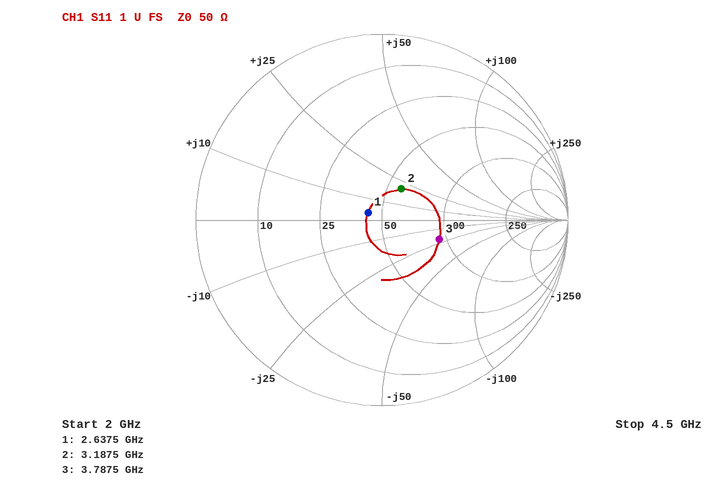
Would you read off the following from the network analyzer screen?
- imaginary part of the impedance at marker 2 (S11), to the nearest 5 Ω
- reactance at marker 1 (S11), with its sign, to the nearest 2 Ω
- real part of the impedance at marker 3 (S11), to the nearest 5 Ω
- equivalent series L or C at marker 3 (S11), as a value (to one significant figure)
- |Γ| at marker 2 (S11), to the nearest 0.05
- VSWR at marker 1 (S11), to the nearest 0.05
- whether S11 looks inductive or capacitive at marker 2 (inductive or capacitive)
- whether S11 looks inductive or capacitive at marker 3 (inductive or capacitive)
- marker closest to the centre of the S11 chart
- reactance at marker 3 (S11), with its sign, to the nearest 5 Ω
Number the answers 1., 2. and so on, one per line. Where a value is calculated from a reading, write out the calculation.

1. +20 Ω
2. +4 Ω
3. 90 Ω
4. C = 1/(2π × 3.7875 GHz × 20 Ω) ≈ 2 pF
5. 0.20
6. 1.20
7. inductive
8. capacitive
9. marker 1
10. -20 Ω
